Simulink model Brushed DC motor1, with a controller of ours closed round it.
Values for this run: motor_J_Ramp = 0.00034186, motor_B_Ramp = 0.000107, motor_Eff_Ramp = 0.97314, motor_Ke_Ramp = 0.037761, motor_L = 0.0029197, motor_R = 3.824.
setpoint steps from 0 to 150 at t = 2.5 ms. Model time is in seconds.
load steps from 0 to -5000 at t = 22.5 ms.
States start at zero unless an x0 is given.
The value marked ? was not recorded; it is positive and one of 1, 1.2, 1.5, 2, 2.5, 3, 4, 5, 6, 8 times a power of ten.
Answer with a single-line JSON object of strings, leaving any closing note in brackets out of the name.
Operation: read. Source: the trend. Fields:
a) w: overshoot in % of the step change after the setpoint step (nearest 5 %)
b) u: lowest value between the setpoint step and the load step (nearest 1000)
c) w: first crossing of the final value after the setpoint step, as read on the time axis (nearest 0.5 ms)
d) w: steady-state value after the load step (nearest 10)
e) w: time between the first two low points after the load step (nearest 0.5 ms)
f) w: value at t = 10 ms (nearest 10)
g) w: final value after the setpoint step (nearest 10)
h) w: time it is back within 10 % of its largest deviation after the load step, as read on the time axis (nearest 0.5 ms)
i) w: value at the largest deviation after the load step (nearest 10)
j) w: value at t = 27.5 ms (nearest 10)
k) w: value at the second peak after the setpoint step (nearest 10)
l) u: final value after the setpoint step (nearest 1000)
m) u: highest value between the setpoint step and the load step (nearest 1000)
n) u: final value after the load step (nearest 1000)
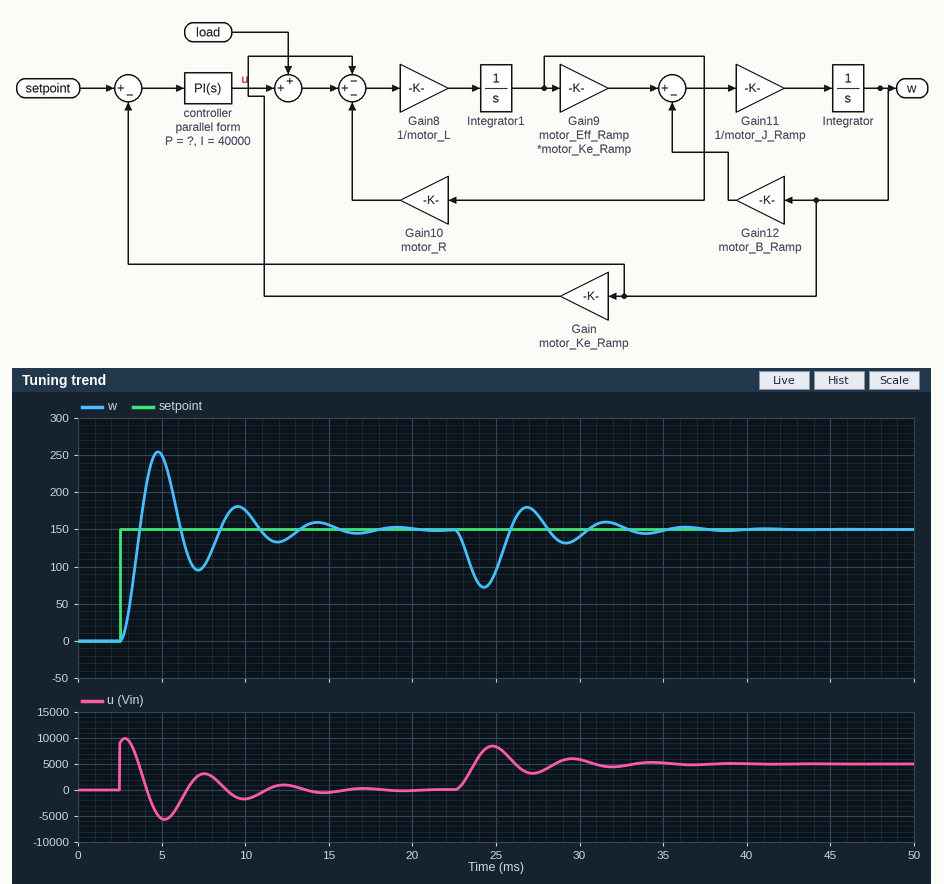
{"w: overshoot in % of the step change after the setpoint step": "70 %", "u: lowest value between the setpoint step and the load step": "-6000", "w: first crossing of the final value after the setpoint step, as read on the time axis": "3.5 ms", "w: steady-state value after the load step": "150", "w: time between the first two low points after the load step": "5.0 ms", "w: value at t = 10 ms": "180", "w: final value after the setpoint step": "150", "w: time it is back within 10 % of its largest deviation after the load step, as read on the time axis": "32.0 ms", "w: value at the largest deviation after the load step": "70", "w: value at t = 27.5 ms": "170", "w: value at the second peak after the setpoint step": "180", "u: final value after the setpoint step": "0", "u: highest value between the setpoint step and the load step": "10000", "u: final value after the load step": "5000"}
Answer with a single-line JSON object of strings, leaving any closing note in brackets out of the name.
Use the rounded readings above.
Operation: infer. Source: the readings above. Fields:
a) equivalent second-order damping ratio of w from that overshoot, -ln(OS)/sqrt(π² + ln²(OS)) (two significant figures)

{"equivalent second-order damping ratio of w from that overshoot, -ln(OS)/sqrt(π² + ln²(OS))": "0.11"}
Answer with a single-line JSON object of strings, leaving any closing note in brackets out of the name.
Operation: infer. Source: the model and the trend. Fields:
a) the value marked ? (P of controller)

{"the value marked ?": "60"}
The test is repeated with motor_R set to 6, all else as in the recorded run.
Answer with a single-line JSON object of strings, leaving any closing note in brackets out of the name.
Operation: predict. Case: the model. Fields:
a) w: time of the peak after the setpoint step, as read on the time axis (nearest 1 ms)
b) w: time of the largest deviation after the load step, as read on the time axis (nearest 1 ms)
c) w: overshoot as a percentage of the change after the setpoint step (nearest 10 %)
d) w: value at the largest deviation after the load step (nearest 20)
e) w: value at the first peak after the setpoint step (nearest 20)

{"w: time of the peak after the setpoint step, as read on the time axis": "5 ms", "w: time of the largest deviation after the load step, as read on the time axis": "24 ms", "w: overshoot as a percentage of the change after the setpoint step": "50 %", "w: value at the largest deviation after the load step": "80", "w: value at the first peak after the setpoint step": "220"}
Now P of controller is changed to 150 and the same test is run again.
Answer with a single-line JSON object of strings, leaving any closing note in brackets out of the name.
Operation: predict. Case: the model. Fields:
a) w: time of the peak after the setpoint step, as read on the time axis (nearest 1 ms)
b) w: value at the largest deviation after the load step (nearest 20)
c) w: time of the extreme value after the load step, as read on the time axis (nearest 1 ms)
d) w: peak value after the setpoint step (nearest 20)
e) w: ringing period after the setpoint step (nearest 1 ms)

{"w: time of the peak after the setpoint step, as read on the time axis": "4 ms", "w: value at the largest deviation after the load step": "100", "w: time of the extreme value after the load step, as read on the time axis": "24 ms", "w: peak value after the setpoint step": "240", "w: ringing period after the setpoint step": "3 ms"}
